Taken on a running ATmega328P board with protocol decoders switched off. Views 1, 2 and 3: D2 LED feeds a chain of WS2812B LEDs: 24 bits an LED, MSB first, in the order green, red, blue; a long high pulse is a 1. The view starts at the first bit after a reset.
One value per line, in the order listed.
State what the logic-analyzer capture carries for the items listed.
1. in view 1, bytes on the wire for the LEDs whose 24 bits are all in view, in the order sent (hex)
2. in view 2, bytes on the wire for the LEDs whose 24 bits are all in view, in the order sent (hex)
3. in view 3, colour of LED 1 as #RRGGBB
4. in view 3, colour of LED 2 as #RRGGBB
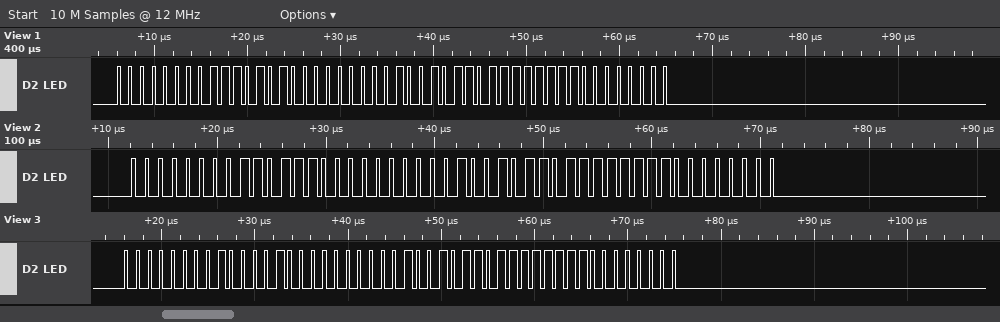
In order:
00 EA 00 96 FF 00
00 DC 00 96 FF 00
#840000
#FF9600
